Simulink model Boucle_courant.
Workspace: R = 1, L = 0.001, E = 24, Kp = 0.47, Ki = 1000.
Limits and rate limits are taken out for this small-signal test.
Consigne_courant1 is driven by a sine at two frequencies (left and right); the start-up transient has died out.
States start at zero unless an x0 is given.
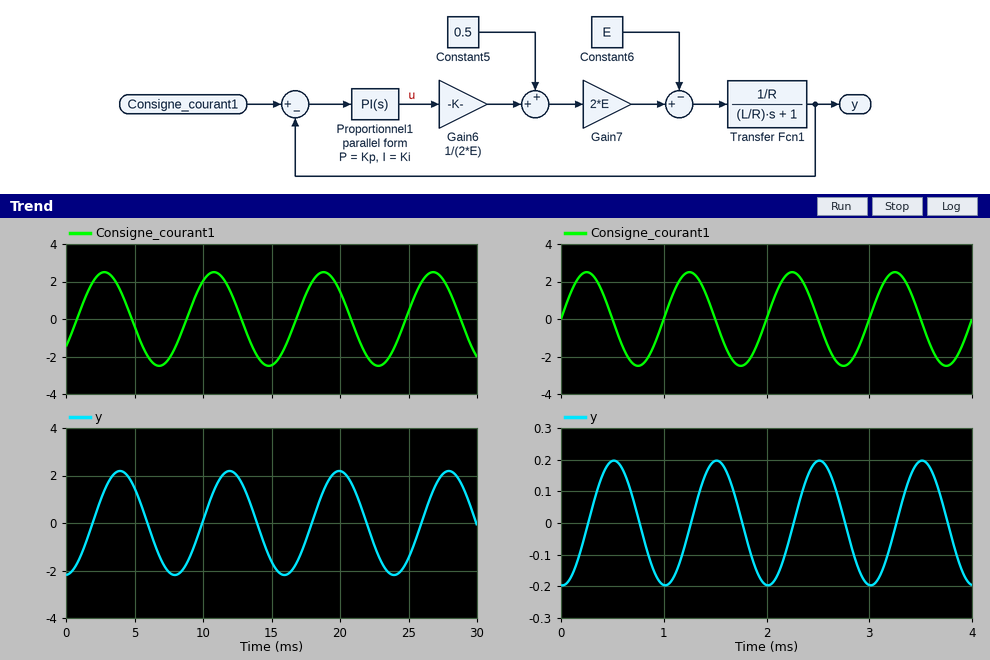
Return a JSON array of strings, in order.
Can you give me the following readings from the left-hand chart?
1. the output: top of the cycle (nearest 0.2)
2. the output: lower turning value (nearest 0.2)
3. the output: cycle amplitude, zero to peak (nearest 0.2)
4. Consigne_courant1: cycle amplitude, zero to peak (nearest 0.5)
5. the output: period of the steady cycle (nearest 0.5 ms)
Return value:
["2.2", "-2.2", "2.2", "2.5", "8.0 ms"]
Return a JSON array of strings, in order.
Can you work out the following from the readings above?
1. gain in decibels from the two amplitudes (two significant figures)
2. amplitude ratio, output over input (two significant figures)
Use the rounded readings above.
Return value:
["-1.1 dB", "0.88"]
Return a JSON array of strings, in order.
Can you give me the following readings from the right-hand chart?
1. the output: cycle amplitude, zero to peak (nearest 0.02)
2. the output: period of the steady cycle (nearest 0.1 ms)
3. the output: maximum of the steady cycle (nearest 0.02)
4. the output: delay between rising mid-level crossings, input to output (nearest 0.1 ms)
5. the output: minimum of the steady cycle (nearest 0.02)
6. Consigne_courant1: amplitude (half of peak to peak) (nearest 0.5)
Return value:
["0.20", "1.0 ms", "0.20", "0.3 ms", "-0.20", "2.5"]
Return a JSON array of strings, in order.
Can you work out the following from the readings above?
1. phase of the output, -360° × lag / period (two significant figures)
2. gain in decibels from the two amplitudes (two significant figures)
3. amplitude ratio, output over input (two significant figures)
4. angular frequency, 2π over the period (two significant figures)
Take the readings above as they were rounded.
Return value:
["-110°", "-22 dB", "0.080", "6.3 rad/ms"]
